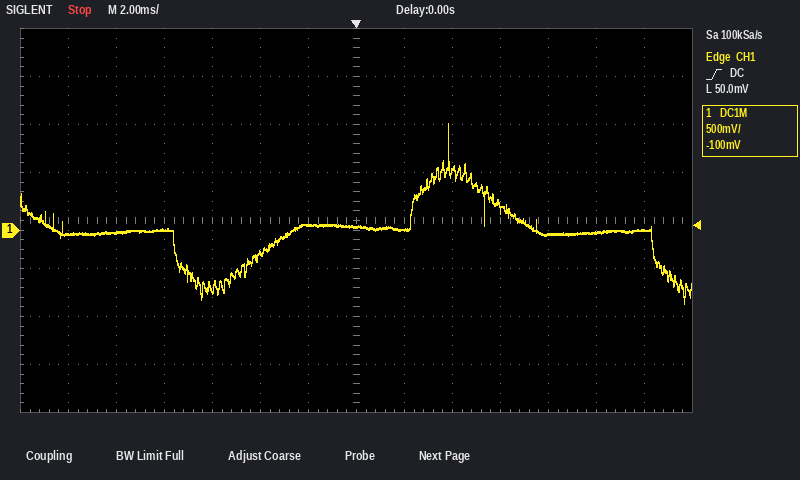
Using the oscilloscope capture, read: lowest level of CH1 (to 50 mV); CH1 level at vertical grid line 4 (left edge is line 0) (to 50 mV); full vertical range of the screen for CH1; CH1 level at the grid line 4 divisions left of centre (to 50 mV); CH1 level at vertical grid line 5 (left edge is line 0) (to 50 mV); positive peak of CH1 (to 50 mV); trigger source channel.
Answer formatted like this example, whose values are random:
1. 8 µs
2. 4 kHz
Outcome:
1. -750 mV
2. -600 mV
3. 4 V
4. 0 mV
5. -250 mV
6. 1.10 V
7. CH1
